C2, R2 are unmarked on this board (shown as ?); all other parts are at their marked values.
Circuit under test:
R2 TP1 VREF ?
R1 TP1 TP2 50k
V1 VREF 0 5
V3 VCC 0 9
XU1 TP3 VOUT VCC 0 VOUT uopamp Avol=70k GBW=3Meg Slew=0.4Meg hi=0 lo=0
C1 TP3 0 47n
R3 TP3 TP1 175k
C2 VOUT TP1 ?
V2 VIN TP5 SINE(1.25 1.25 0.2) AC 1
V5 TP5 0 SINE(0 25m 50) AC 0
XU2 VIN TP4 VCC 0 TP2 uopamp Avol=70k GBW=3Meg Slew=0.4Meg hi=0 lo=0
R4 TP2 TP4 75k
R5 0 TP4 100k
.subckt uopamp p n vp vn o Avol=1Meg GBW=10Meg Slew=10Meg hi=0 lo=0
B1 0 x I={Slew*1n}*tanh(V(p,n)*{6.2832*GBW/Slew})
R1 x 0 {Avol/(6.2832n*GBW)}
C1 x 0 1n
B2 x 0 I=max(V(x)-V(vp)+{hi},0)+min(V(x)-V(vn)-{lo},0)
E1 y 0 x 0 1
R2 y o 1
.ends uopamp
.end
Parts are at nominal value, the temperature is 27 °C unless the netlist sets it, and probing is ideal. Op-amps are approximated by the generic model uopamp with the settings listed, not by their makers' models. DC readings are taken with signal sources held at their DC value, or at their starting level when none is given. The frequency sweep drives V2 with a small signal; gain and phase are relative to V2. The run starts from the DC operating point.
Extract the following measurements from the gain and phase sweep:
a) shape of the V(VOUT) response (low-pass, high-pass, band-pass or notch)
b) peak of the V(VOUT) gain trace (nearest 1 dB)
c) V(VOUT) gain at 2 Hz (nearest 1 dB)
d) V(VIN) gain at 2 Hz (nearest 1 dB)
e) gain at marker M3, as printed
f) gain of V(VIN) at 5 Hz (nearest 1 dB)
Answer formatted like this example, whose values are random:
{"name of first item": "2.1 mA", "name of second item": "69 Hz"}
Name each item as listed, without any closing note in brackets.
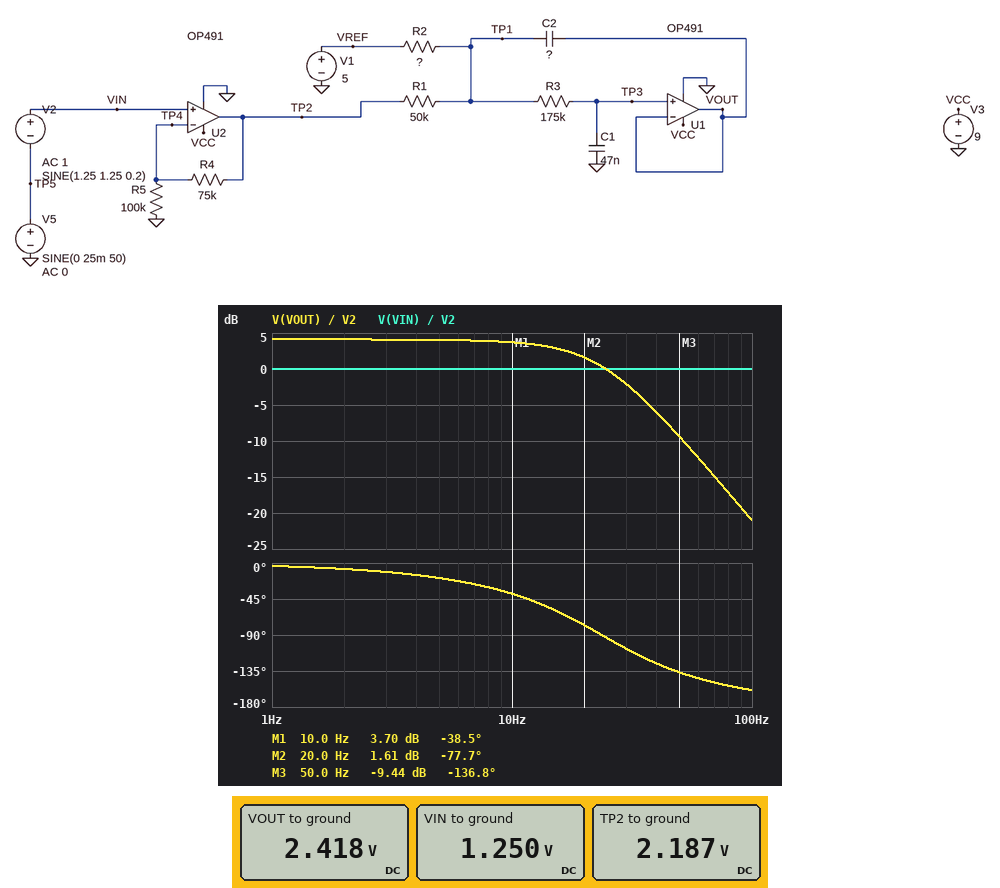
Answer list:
{"shape of the V(VOUT) response": "low-pass", "peak of the V(VOUT) gain trace": "4 dB", "V(VOUT) gain at 2 Hz": "4 dB", "V(VIN) gain at 2 Hz": "0 dB", "gain at marker M3, as printed": "-9.44 dB", "gain of V(VIN) at 5 Hz": "0 dB"}
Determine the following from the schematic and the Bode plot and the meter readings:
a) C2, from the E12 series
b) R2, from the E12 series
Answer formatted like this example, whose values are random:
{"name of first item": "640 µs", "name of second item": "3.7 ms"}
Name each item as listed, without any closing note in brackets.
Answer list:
{"C2, from the E12 series": "120 nF", "R2, from the E12 series": "560 kΩ"}
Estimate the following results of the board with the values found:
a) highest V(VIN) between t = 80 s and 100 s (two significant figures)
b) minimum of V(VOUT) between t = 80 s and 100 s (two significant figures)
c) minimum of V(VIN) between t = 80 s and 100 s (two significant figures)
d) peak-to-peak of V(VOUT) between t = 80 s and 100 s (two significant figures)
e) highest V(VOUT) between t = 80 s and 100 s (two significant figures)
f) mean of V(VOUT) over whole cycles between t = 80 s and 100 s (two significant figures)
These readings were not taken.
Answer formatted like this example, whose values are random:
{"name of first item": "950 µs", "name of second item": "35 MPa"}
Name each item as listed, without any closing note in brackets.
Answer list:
{"highest V(VIN) between t = 80 s and 100 s": "2.5 V", "minimum of V(VOUT) between t = 80 s and 100 s": "420 mV", "minimum of V(VIN) between t = 80 s and 100 s": "-25 mV", "peak-to-peak of V(VOUT) between t = 80 s and 100 s": "4.0 V", "highest V(VOUT) between t = 80 s and 100 s": "4.4 V", "mean of V(VOUT) over whole cycles between t = 80 s and 100 s": "2.4 V"}
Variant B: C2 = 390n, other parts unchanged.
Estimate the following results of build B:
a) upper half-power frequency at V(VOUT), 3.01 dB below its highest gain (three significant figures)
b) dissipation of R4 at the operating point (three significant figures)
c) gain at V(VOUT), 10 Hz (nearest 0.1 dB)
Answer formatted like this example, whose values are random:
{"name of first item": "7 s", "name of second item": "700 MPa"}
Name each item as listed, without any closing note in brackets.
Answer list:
{"upper half-power frequency at V(VOUT), 3.01 dB below its highest gain": "15.6 Hz", "dissipation of R4 at the operating point": "11.7 µW", "gain at V(VOUT), 10 Hz": "6.3 dB"}
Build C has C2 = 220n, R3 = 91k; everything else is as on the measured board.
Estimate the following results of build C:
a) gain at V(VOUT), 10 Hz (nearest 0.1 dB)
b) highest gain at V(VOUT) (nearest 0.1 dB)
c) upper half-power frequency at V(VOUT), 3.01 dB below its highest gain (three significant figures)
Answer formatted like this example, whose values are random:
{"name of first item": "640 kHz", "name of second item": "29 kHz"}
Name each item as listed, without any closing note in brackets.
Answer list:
{"gain at V(VOUT), 10 Hz": "4.8 dB", "highest gain at V(VOUT)": "5.5 dB", "upper half-power frequency at V(VOUT), 3.01 dB below its highest gain": "28.4 Hz"}
